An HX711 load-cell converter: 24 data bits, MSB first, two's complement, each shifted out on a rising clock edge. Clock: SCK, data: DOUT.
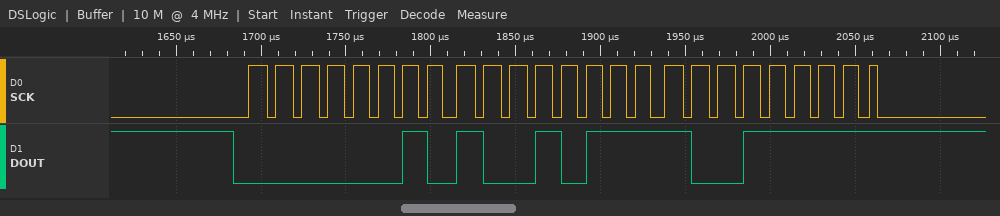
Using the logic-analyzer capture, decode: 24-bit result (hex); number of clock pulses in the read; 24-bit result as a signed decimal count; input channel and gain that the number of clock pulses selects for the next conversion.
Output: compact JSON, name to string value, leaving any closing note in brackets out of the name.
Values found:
{"24-bit result": "0x02979F", "number of clock pulses in the read": "25", "24-bit result as a signed decimal count": "169887", "input channel and gain that the number of clock pulses selects for the next conversion": "channel A, gain 128"}
